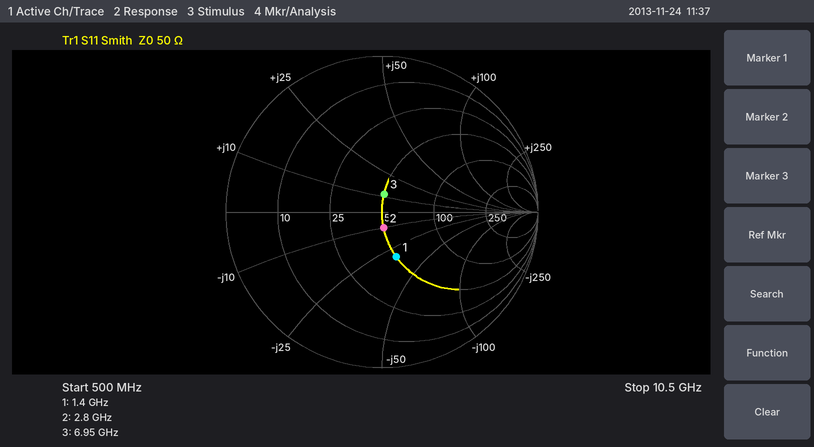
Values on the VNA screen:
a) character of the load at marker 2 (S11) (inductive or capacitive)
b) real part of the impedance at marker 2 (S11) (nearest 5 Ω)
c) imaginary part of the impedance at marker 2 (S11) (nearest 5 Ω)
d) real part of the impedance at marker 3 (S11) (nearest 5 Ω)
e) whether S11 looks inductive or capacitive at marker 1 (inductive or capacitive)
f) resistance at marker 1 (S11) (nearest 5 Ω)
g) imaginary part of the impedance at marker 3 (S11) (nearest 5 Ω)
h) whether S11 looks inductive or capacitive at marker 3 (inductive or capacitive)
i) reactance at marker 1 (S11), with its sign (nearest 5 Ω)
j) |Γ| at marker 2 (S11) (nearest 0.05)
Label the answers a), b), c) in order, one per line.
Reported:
a) capacitive
b) 50 Ω
c) -10 Ω
d) 50 Ω
e) capacitive
f) 50 Ω
g) +10 Ω
h) inductive
i) -30 Ω
j) 0.10
